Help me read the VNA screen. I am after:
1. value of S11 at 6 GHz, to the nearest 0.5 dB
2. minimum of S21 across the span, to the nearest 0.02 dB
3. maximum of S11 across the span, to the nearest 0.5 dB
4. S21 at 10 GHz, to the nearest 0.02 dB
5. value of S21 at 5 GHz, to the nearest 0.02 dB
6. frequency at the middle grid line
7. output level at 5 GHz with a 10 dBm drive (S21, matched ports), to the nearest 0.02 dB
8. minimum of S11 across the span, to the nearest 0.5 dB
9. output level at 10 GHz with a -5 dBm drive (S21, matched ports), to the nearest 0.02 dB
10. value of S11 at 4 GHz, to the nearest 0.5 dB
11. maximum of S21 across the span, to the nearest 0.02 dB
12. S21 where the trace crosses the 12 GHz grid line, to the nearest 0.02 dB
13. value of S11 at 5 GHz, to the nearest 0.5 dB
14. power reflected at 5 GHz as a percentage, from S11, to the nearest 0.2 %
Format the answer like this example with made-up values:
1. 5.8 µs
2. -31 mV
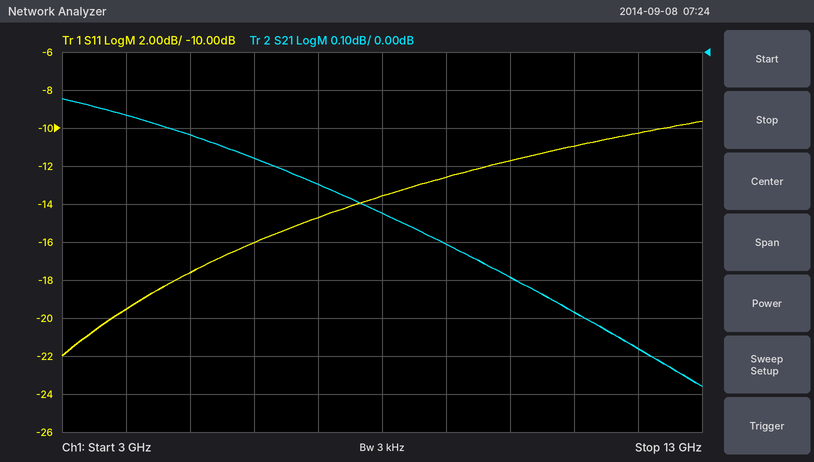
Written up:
1. -16.0 dB
2. -0.88 dB
3. -9.5 dB
4. -0.60 dB
5. -0.22 dB
6. 8 GHz
7. 9.78 dBm
8. -22.0 dB
9. -5.60 dBm
10. -19.5 dB
11. -0.12 dB
12. -0.78 dB
13. -17.5 dB
14. 1.8 %
